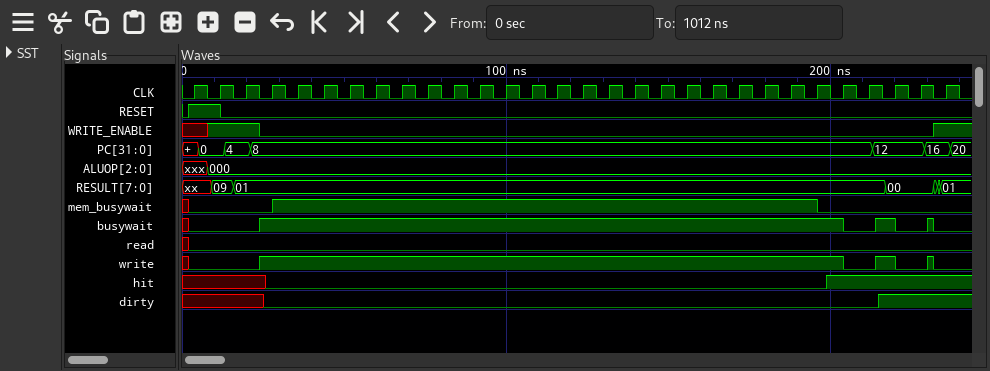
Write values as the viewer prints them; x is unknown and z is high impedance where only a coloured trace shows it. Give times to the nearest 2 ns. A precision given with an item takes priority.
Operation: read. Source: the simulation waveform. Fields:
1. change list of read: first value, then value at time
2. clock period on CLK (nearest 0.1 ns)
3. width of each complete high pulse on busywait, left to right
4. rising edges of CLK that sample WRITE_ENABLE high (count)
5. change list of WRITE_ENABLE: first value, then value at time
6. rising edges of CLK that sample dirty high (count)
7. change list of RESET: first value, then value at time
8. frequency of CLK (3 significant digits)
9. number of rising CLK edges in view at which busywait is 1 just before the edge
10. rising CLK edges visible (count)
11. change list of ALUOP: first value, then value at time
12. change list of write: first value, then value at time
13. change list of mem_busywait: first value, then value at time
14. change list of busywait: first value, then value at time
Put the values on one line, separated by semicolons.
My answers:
x, 0 at 2 ns; 8 ns; 180 ns, 6 ns, 2 ns; 3; x, 1 at 8 ns, 0 at 24 ns, 1 at 232 ns; 3; 0, 1 at 2 ns, 0 at 12 ns; 125 MHz; 24; 30; xxx, 000 at 8 ns; x, 0 at 2 ns, 1 at 24 ns, 0 at 204 ns, 1 at 214 ns, 0 at 220 ns, 1 at 230 ns, 0 at 232 ns; x, 0 at 2 ns, 1 at 28 ns, 0 at 196 ns; x, 0 at 2 ns, 1 at 24 ns, 0 at 204 ns, 1 at 214 ns, 0 at 220 ns, 1 at 230 ns, 0 at 232 ns
